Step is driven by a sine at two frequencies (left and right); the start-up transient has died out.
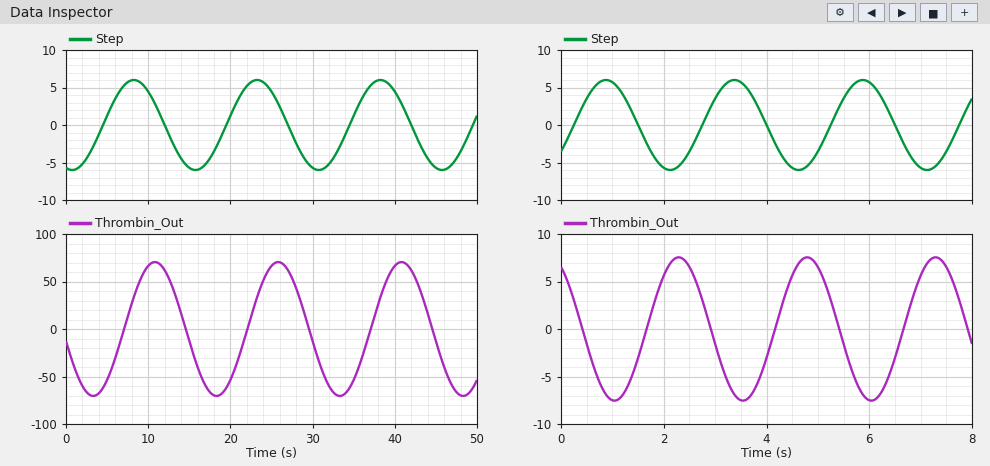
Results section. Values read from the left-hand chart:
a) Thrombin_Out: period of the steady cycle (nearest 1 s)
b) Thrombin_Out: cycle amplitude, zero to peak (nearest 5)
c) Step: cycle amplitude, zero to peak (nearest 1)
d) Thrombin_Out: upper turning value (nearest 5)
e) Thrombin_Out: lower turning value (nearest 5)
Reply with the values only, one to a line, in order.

15 s
70
6
70
-70
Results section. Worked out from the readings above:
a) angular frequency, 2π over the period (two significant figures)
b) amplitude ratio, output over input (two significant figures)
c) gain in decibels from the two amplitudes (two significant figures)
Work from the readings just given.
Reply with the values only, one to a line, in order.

0.42 rad/s
12
21 dB
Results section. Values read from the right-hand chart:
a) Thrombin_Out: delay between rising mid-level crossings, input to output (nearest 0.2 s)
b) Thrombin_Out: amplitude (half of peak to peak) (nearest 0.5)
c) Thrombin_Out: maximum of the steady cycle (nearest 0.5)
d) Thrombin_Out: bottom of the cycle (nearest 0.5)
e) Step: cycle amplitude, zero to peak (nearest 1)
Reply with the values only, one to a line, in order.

1.4 s
7.5
7.5
-7.5
6
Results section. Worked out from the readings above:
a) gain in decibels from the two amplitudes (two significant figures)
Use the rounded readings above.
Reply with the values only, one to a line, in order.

1.9 dB
